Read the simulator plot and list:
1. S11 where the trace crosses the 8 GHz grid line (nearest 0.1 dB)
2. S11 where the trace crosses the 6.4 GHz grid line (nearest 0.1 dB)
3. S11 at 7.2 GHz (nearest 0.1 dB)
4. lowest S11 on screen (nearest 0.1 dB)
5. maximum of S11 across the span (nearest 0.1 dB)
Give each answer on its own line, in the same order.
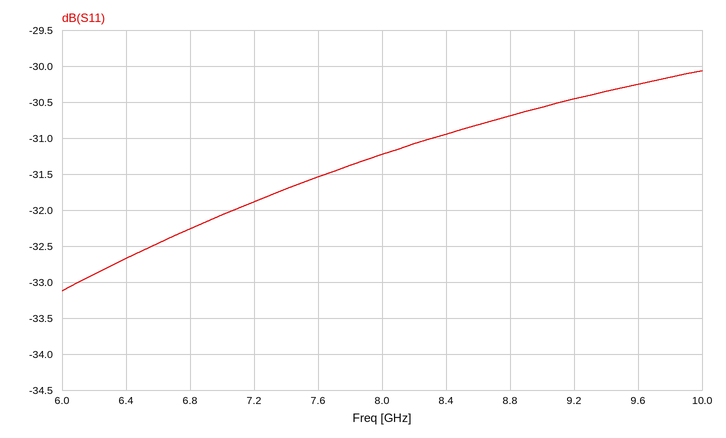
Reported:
-31.2 dB
-32.7 dB
-31.9 dB
-33.1 dB
-30.1 dB
